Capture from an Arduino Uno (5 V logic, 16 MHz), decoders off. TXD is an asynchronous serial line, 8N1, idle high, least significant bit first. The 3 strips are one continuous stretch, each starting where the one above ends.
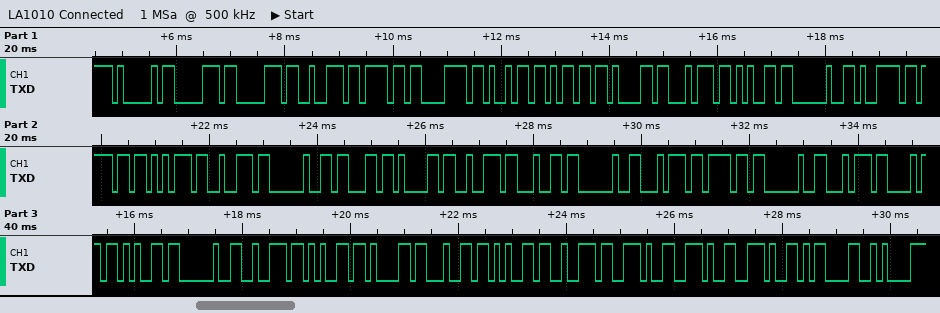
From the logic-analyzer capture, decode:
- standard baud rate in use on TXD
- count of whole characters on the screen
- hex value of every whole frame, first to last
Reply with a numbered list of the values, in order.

1. 9600 baud
2. 40
3. 0x41 0x70 0x70 0x72 0x6F 0x78 0x69 0x6D 0x61 0x74 0x65 0x20 0x79 0x6F 0x75 0x72 0x20 0x63 0x61 0x72 0x64 0x20 0x74 0x6F 0x20 0x74 0x68 0x65 0x20 0x72 0x65 0x61 0x64 0x65 0x72 0x2E 0x2E 0x2E 0x0D 0x0A
